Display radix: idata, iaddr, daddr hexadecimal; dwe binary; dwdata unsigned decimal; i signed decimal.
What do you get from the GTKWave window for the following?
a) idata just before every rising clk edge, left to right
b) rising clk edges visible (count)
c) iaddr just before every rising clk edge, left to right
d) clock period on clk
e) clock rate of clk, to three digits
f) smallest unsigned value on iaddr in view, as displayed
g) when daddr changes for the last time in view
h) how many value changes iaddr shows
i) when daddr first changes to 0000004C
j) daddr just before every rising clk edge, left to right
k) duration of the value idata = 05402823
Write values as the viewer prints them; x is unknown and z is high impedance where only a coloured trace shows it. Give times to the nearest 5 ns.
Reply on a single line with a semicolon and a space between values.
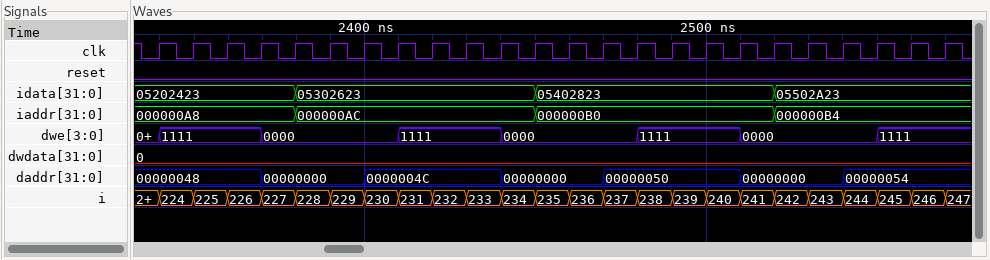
05202423, 05202423, 05202423, 05202423, 05202423, 05302623, 05302623, 05302623, 05302623, 05302623, 05302623, 05302623, 05402823, 05402823, 05402823, 05402823, 05402823, 05402823, 05402823, 05502A23, 05502A23, 05502A23, 05502A23, 05502A23; 24; 000000A8, 000000A8, 000000A8, 000000A8, 000000A8, 000000AC, 000000AC, 000000AC, 000000AC, 000000AC, 000000AC, 000000AC, 000000B0, 000000B0, 000000B0, 000000B0, 000000B0, 000000B0, 000000B0, 000000B4, 000000B4, 000000B4, 000000B4, 000000B4; 10 ns; 100 MHz; 000000A8; 2540 ns; 3; 2400 ns; 00000048, 00000048, 00000048, 00000048, 00000000, 00000000, 00000000, 0000004C, 0000004C, 0000004C, 0000004C, 00000000, 00000000, 00000000, 00000050, 00000050, 00000050, 00000050, 00000000, 00000000, 00000000, 00000054, 00000054, 00000054; 70 ns
